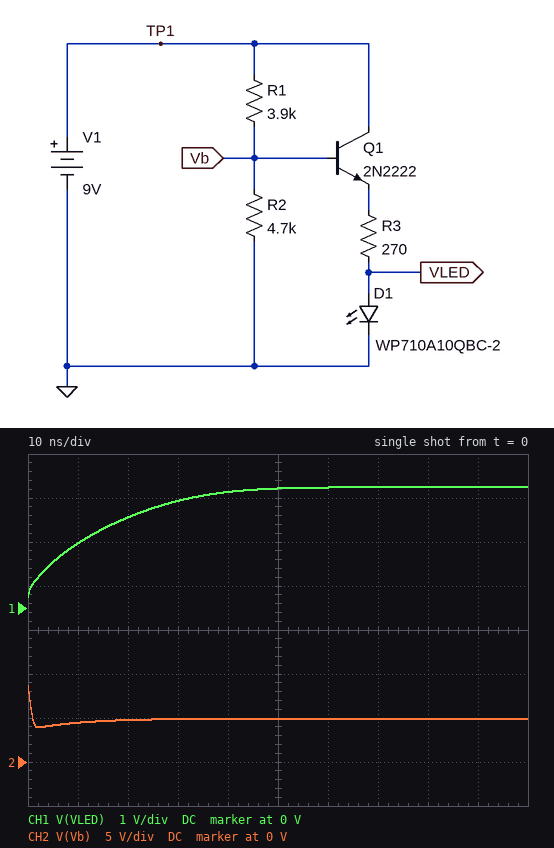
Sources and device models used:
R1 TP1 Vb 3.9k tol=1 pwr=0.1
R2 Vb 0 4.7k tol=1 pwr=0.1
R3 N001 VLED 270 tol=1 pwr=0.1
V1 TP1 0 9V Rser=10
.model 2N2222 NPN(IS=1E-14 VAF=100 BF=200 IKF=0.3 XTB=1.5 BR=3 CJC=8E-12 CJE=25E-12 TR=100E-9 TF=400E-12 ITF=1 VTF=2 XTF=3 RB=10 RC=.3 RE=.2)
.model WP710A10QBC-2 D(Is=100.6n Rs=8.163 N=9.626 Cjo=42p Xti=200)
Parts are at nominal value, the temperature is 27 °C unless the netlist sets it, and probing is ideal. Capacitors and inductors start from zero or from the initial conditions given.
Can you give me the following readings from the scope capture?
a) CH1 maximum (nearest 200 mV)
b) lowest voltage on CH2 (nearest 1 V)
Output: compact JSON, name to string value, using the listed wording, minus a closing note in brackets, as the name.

{"CH1 maximum": "2.8 V", "lowest voltage on CH2": "4 V"}
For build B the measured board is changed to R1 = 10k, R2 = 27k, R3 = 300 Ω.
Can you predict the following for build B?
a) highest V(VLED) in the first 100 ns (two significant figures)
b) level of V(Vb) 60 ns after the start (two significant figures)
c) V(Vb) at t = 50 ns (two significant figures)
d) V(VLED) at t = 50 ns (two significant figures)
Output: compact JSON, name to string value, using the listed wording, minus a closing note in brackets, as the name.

{"highest V(VLED) in the first 100 ns": "2.9 V", "level of V(Vb) 60 ns after the start": "5.9 V", "V(Vb) at t = 50 ns": "5.8 V", "V(VLED) at t = 50 ns": "2.8 V"}
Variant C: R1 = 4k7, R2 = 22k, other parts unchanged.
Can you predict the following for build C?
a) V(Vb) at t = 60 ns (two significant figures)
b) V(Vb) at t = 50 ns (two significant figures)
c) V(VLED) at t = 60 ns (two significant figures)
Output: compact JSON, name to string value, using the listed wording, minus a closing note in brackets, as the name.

{"V(Vb) at t = 60 ns": "6.9 V", "V(Vb) at t = 50 ns": "6.8 V", "V(VLED) at t = 60 ns": "3.0 V"}
